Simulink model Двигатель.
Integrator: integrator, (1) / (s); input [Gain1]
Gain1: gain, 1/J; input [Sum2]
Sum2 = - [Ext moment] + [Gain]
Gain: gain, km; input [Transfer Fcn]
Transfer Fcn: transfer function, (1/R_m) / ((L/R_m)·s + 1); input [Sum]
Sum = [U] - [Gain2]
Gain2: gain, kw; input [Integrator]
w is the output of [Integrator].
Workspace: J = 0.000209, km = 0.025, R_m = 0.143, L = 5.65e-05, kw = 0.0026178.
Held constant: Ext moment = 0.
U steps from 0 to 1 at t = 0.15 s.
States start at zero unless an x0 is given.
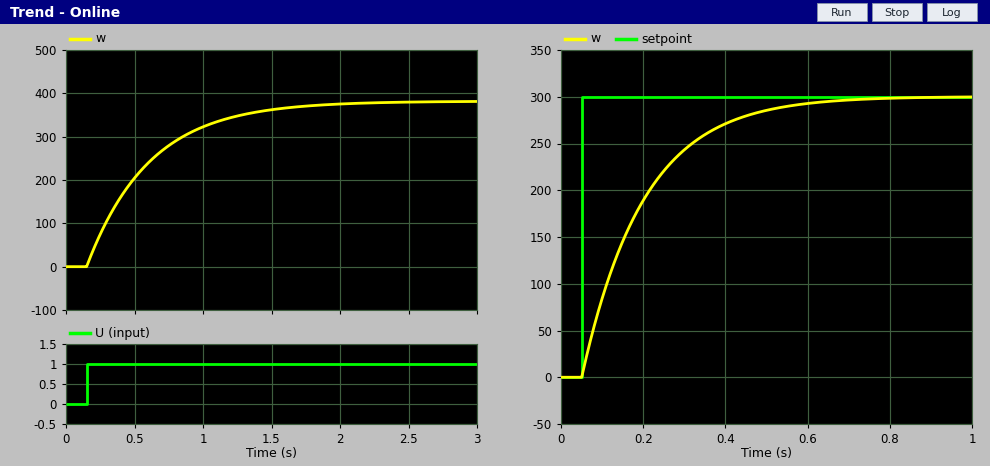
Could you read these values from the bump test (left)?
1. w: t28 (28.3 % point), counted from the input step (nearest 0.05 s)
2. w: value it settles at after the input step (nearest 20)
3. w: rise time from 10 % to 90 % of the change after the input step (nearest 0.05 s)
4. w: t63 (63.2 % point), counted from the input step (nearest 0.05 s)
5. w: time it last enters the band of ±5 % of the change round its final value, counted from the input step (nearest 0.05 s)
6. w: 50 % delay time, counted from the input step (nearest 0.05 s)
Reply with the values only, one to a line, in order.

0.15 s
380
1.00 s
0.45 s
1.35 s
0.30 s
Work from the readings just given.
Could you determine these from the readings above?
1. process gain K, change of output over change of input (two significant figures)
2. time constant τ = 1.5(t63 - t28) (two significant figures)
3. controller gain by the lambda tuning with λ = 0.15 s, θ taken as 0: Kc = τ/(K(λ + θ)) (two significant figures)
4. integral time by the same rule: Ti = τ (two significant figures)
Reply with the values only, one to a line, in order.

380
0.45 s
0.0079
0.45 s
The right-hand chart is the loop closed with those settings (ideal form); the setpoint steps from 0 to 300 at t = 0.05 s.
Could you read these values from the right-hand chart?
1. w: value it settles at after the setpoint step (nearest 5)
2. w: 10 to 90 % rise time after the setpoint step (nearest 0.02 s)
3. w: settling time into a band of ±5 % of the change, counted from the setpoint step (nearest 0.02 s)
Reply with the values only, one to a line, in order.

300
0.32 s
0.44 s
